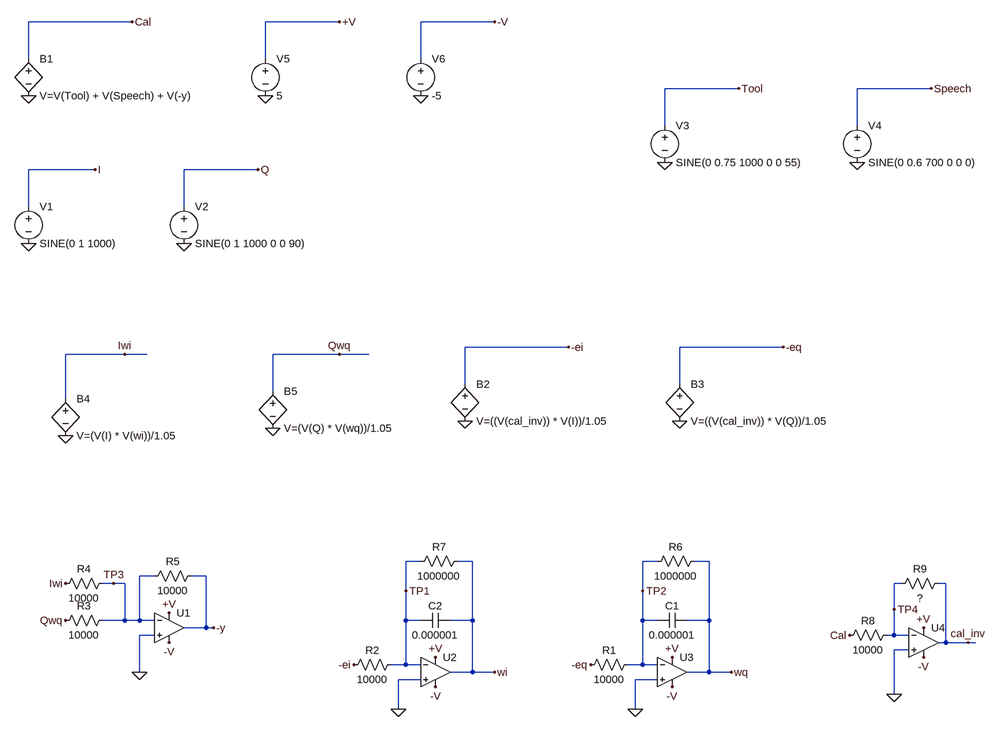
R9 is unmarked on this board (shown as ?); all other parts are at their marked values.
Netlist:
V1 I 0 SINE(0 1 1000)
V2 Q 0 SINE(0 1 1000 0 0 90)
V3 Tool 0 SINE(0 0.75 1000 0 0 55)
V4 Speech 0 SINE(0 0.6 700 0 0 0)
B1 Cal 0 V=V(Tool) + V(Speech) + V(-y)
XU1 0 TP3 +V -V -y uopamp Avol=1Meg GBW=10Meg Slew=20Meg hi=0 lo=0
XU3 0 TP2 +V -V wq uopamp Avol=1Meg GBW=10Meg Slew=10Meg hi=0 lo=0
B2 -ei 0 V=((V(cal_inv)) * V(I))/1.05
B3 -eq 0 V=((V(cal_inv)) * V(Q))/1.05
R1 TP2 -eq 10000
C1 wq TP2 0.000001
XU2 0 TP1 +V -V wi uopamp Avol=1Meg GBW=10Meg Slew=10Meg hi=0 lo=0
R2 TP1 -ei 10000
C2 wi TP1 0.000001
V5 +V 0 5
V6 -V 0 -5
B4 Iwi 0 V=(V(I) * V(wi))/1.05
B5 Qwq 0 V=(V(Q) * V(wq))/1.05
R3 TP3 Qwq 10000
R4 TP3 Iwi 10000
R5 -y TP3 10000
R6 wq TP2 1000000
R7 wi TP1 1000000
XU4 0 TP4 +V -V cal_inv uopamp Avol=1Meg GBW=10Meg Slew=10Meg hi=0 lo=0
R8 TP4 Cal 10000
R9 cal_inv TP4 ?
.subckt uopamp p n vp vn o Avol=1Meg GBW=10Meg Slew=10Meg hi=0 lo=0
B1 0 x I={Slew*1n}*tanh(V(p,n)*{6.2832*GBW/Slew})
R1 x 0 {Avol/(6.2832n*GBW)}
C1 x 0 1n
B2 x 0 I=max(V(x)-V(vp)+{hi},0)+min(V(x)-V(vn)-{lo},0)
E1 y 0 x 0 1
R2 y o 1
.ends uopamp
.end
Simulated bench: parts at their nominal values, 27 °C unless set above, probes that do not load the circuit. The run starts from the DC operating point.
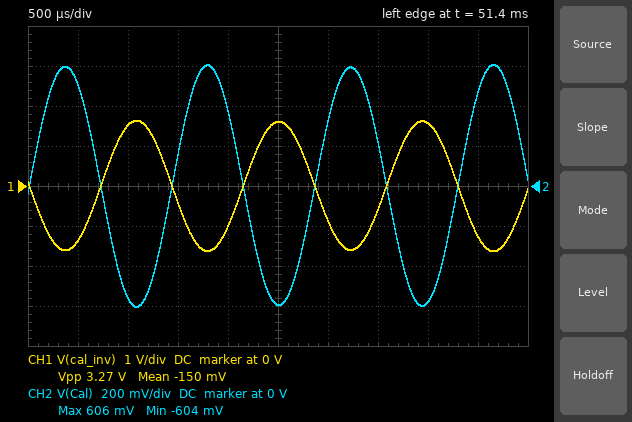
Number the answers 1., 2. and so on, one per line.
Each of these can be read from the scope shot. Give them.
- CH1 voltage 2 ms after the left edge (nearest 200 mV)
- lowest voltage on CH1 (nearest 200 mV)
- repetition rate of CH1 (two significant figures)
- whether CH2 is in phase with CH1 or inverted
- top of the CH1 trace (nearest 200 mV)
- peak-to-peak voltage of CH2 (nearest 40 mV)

1. -1.0 V
2. -1.6 V
3. 700 Hz
4. inverted
5. 1.6 V
6. 1.20 V
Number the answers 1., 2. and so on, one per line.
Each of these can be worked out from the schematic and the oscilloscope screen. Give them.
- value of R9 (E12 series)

1. 27 kΩ
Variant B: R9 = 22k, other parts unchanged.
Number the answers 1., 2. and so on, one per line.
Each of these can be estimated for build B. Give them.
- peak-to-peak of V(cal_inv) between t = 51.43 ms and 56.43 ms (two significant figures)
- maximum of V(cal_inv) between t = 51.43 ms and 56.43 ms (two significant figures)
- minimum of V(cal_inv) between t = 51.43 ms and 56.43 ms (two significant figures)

1. 2.7 V
2. 1.3 V
3. -1.3 V
